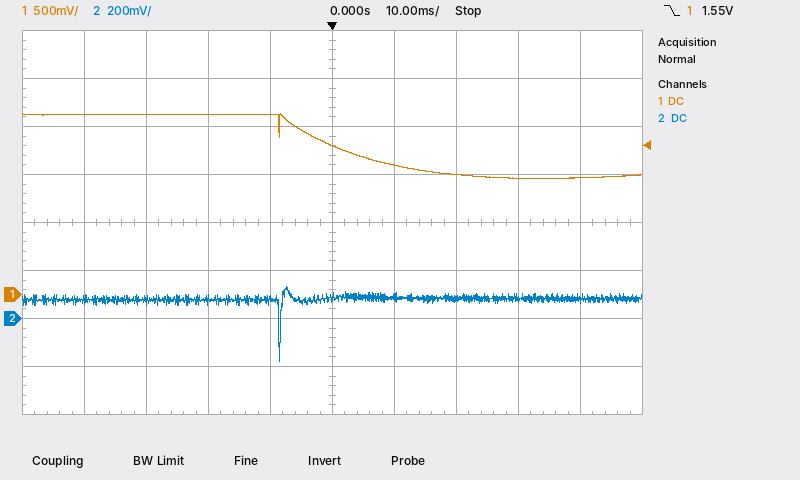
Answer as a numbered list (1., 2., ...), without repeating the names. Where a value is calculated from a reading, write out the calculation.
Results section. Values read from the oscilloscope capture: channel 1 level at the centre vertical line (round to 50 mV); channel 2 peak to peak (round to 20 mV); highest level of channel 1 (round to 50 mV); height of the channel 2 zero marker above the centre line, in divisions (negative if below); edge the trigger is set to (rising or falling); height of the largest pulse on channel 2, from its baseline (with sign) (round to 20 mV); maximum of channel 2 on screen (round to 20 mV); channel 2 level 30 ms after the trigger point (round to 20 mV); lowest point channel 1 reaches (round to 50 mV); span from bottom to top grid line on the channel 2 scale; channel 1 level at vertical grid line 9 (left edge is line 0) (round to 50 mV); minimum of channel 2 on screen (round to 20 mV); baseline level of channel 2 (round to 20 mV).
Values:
1. 1.55 V
2. 140 mV − (-180 mV) = 320 mV
3. 1.90 V
4. -2.0 div
5. falling
6. -180 mV − (80 mV) = -260 mV
7. 140 mV
8. 80 mV
9. 1.20 V
10. 1.6 V
11. 1.20 V
12. -180 mV
13. 80 mV
